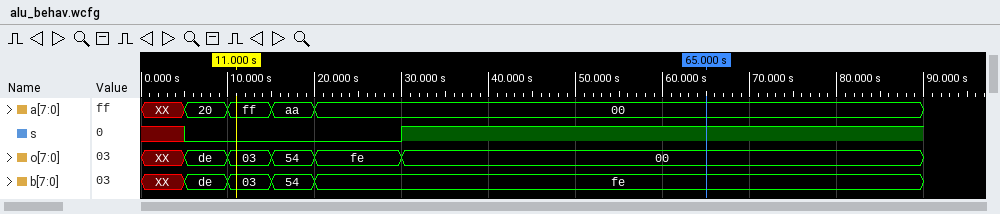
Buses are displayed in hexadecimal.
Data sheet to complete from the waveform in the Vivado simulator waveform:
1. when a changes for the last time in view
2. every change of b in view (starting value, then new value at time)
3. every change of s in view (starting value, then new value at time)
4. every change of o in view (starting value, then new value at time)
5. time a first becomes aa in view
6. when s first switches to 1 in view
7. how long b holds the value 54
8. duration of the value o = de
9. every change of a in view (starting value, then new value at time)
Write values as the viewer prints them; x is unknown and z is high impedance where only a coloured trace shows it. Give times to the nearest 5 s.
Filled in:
20 s
XX, de at 5 s, 03 at 10 s, 54 at 15 s, fe at 20 s
x, 0 at 5 s, 1 at 30 s
XX, de at 5 s, 03 at 10 s, 54 at 15 s, fe at 20 s, 00 at 30 s
15 s
30 s
5 s
5 s
XX, 20 at 5 s, ff at 10 s, aa at 15 s, 00 at 20 s
